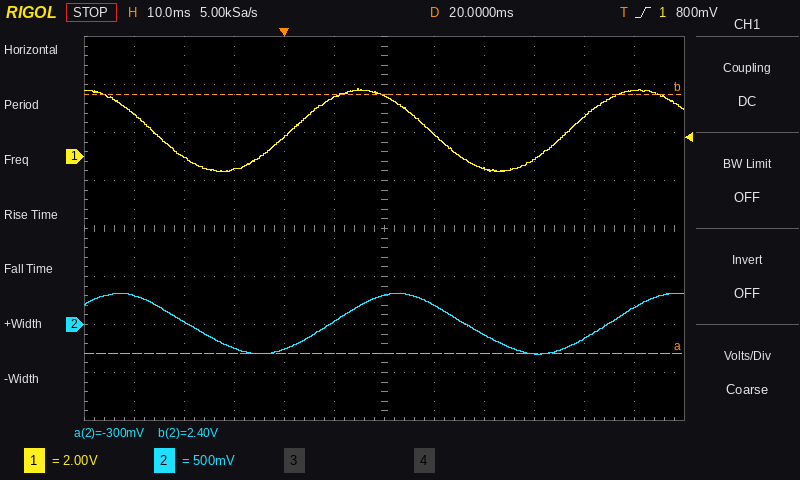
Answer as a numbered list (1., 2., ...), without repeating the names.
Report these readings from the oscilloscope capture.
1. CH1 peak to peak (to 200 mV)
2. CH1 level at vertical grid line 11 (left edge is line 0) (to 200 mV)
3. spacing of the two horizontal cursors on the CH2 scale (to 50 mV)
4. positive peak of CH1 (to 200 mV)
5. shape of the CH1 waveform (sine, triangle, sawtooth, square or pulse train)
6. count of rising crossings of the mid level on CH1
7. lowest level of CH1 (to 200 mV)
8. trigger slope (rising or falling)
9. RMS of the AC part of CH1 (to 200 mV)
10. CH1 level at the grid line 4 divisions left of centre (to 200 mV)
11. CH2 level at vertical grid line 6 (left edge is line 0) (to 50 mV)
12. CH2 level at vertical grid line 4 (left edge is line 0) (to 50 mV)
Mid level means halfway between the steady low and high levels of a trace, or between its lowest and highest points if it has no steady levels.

1. 3.4 V
2. 2.8 V
3. 2.70 V
4. 2.8 V
5. sine
6. 2
7. -600 mV
8. rising
9. 1.2 V
10. 0.0 V
11. 300 mV
12. -250 mV
